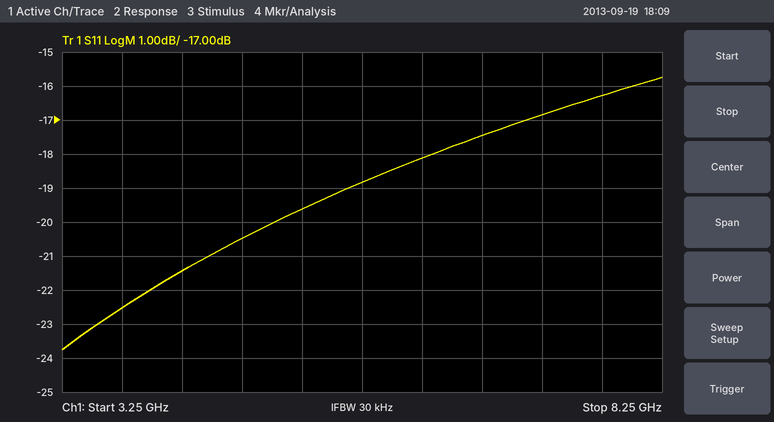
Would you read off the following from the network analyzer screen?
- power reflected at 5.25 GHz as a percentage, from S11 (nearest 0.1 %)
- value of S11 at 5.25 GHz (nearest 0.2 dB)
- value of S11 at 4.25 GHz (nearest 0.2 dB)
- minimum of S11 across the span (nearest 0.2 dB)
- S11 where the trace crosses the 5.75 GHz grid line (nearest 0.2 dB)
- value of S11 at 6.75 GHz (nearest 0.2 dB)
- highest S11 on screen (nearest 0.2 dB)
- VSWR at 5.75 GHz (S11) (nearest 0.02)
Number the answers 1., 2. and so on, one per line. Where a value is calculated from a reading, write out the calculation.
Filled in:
1. 10^(-19.6/10) ≈ 1.1 %
2. -19.6 dB
3. -21.4 dB
4. -23.8 dB
5. -18.8 dB
6. -17.4 dB
7. -15.8 dB
8. |Γ| = 10^(-18.8/20) = 0.1148; VSWR = (1 + 0.1148)/(1 − 0.1148) ≈ 1.26
